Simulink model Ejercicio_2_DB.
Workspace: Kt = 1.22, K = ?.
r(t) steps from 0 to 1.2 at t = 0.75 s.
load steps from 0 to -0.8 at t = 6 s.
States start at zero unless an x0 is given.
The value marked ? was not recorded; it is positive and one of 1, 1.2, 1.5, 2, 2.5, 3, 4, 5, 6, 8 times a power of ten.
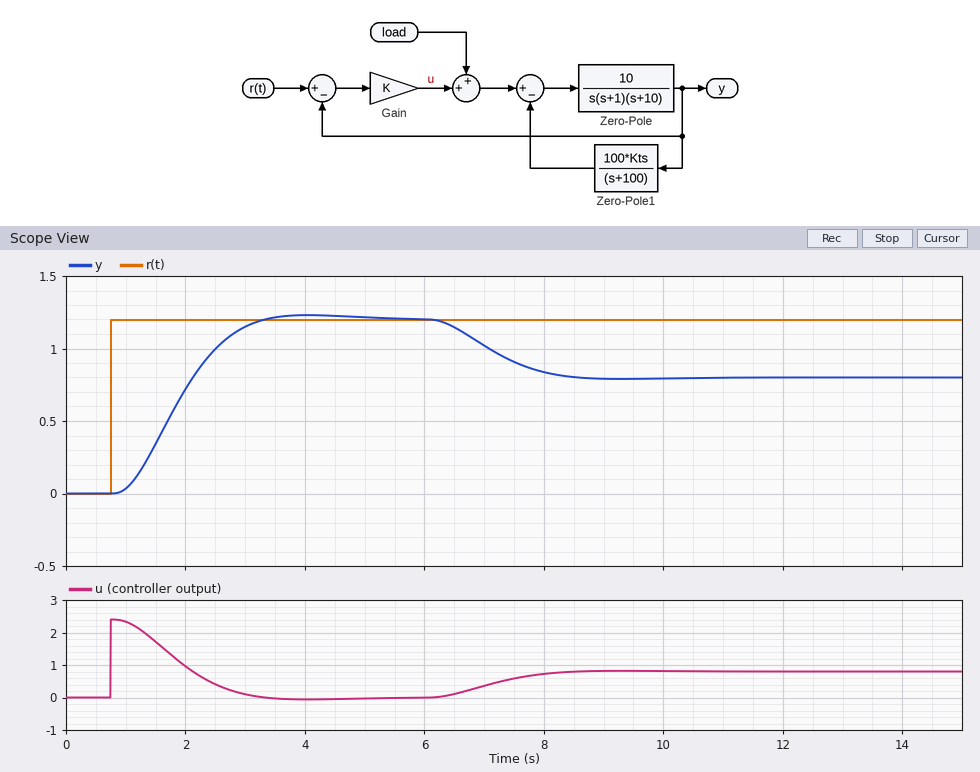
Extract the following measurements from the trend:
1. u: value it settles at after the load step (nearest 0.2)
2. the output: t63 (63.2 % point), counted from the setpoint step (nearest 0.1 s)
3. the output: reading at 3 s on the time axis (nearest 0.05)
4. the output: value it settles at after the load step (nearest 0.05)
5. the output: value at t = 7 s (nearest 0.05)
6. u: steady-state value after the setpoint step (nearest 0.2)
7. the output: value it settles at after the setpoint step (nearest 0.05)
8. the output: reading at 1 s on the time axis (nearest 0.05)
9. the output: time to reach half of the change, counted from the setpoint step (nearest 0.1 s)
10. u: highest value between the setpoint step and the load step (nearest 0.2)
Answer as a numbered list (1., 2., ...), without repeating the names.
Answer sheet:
1. 0.8
2. 1.3 s
3. 1.15
4. 0.80
5. 1.00
6. 0.0
7. 1.20
8. 0.05
9. 1.1 s
10. 2.4
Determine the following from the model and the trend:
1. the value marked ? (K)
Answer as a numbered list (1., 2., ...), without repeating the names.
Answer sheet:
1. 2
